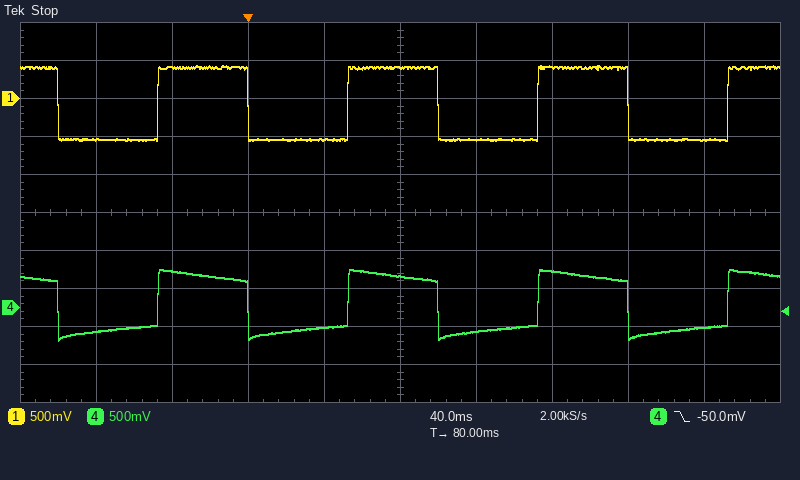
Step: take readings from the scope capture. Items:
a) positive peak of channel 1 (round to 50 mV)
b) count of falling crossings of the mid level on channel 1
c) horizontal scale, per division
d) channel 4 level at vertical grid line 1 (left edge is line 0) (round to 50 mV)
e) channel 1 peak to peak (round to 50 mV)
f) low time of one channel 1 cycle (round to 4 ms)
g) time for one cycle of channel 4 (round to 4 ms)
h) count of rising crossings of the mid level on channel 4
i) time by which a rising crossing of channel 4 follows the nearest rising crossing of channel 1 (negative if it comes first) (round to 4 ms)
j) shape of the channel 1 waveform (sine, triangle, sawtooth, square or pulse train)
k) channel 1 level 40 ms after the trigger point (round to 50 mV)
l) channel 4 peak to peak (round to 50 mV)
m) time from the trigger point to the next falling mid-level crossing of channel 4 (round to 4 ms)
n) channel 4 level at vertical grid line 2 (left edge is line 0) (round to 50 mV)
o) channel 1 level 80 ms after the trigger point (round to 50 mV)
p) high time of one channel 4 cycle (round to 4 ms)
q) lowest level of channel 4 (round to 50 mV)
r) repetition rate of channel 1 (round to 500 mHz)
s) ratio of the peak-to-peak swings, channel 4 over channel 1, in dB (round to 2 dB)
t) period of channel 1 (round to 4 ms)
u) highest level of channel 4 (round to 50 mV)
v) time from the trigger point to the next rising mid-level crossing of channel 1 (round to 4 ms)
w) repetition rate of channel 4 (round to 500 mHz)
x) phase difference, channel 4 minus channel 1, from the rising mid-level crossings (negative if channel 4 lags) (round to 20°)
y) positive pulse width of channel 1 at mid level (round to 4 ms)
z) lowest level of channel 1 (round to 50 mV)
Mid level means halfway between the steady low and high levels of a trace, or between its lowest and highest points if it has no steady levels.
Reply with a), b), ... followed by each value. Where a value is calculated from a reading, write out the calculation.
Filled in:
a) 450 mV
b) 4
c) 40 ms
d) -300 mV
e) 450 mV − (-550 mV) = 1.00 V
f) 52 ms
g) 100 ms
h) 4
i) 0 ms
j) square
k) -550 mV
l) 500 mV − (-450 mV) = 950 mV
m) 100 ms
n) 500 mV
o) 400 mV
p) 48 ms
q) -450 mV
r) 1 / 100 ms ≈ 10.0 Hz
s) 20 log10(950 mV / 1.00 V) ≈ 0 dB
t) 100 ms
u) 500 mV
v) 52 ms
w) 1 / 100 ms ≈ 10.0 Hz
x) −360° × (0 ms) / 100 ms ≈ 0°
y) 48 ms
z) -550 mV
